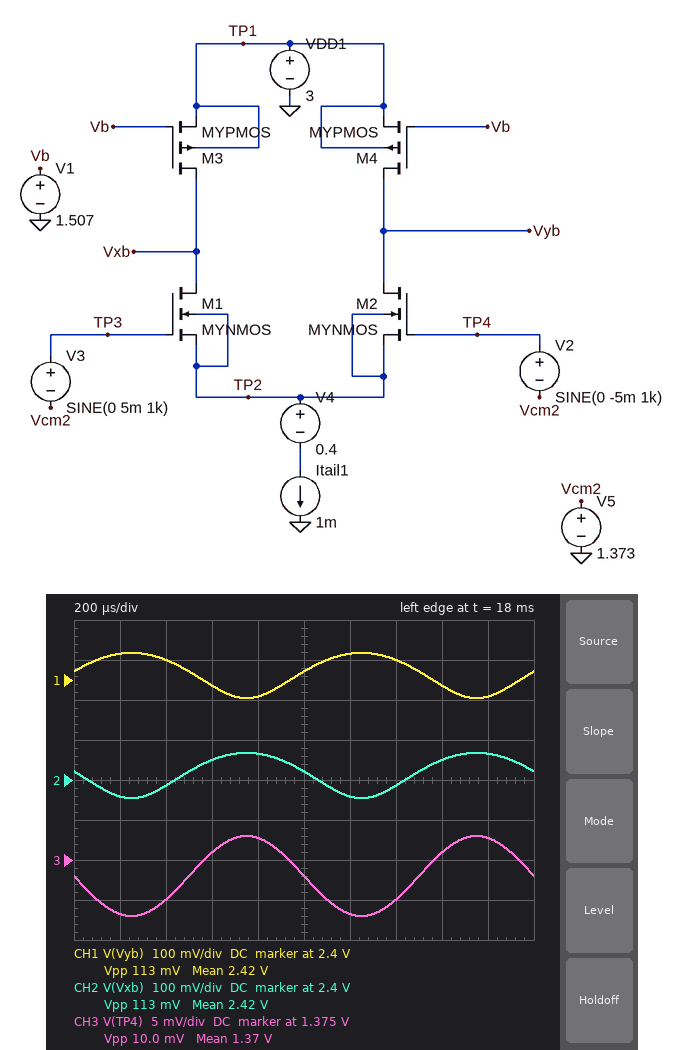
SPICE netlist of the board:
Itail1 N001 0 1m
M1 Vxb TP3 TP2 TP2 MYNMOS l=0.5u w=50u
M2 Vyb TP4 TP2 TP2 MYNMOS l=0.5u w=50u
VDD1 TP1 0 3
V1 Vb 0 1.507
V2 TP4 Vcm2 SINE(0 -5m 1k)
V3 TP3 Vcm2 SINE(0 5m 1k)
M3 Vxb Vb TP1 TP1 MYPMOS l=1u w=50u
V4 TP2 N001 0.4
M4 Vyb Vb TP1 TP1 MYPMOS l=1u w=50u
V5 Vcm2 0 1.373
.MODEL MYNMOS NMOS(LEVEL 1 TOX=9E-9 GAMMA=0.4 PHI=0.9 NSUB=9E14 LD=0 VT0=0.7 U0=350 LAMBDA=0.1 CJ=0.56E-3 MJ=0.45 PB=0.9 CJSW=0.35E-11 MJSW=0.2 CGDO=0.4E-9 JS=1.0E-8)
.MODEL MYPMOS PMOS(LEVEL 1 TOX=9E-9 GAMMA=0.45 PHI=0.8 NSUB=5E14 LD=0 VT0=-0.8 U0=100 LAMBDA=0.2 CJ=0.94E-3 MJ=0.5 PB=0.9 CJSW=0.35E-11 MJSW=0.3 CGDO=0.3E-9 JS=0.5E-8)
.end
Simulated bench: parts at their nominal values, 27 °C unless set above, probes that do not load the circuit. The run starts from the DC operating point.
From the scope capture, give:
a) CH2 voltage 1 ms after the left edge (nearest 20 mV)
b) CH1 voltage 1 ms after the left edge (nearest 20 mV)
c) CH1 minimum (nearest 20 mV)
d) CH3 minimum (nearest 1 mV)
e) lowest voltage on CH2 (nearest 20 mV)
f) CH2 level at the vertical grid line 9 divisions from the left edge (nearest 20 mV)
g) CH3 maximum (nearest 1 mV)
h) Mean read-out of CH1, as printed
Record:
2.42 V
2.42 V
2.36 V
1.368 V
2.36 V
2.46 V
1.378 V
2.42 V
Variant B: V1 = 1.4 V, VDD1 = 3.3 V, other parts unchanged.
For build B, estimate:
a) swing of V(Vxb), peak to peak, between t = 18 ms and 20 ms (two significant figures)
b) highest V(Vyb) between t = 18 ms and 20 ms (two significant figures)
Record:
22 mV
3.1 V
